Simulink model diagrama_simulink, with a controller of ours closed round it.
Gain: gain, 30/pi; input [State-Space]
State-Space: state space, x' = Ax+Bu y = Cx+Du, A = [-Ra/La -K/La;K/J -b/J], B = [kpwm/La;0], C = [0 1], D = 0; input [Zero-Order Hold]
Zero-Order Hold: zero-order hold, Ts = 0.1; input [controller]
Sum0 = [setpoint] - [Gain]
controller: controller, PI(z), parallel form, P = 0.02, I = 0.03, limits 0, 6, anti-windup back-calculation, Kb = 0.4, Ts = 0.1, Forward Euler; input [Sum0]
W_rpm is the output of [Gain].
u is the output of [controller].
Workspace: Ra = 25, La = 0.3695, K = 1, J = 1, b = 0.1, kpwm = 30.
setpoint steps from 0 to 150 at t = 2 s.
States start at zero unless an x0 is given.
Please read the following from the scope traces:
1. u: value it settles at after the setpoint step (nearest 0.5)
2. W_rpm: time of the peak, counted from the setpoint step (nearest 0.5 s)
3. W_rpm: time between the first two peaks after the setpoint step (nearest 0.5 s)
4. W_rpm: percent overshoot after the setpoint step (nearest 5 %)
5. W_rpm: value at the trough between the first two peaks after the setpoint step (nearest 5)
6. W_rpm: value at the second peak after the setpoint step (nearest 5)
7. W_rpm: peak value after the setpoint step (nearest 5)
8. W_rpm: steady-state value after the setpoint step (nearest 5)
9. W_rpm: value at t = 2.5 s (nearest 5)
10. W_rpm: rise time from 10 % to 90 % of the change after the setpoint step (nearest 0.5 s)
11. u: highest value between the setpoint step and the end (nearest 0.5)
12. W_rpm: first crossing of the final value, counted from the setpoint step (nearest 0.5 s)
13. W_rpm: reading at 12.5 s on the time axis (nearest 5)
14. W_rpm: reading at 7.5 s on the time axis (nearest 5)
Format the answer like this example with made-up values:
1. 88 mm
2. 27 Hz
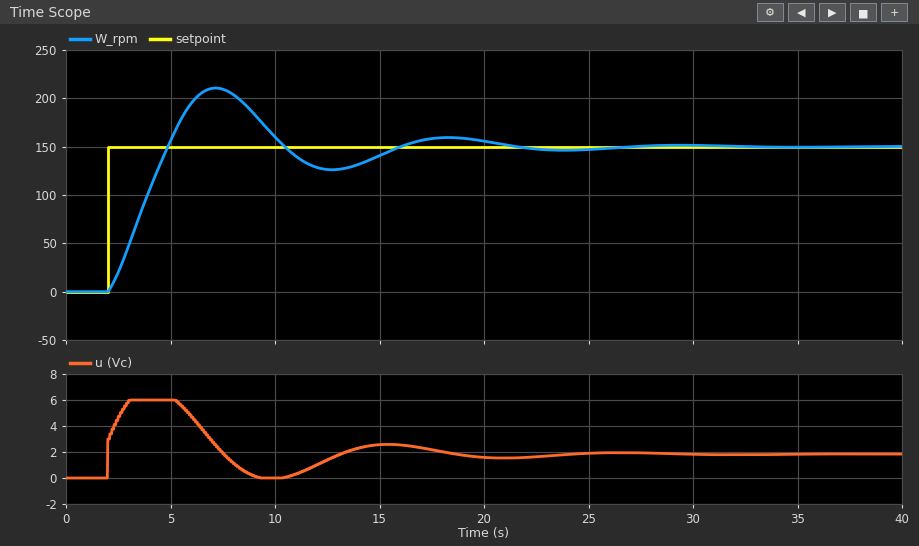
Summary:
1. 2.0
2. 5.0 s
3. 11.0 s
4. 40 %
5. 125
6. 160
7. 210
8. 150
9. 20
10. 2.0 s
11. 6.0
12. 3.0 s
13. 125
14. 210
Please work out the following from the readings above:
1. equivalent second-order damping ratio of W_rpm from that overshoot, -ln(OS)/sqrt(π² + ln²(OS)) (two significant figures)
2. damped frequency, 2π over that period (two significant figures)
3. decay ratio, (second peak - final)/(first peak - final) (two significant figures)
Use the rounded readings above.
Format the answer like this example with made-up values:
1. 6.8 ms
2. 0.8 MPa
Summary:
1. 0.28
2. 0.57 rad/s
3. 0.17
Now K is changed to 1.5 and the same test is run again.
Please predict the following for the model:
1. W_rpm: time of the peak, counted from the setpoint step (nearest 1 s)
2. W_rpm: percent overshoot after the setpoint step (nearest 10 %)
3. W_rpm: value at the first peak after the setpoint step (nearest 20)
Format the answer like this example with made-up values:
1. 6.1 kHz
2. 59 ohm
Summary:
1. 4 s
2. 40 %
3. 200
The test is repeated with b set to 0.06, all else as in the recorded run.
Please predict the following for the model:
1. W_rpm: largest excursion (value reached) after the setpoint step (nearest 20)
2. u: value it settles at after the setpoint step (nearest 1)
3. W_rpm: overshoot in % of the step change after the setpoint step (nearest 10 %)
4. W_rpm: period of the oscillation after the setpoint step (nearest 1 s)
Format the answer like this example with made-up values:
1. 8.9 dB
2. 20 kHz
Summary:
1. 220
2. 1
3. 50 %
4. 12 s
